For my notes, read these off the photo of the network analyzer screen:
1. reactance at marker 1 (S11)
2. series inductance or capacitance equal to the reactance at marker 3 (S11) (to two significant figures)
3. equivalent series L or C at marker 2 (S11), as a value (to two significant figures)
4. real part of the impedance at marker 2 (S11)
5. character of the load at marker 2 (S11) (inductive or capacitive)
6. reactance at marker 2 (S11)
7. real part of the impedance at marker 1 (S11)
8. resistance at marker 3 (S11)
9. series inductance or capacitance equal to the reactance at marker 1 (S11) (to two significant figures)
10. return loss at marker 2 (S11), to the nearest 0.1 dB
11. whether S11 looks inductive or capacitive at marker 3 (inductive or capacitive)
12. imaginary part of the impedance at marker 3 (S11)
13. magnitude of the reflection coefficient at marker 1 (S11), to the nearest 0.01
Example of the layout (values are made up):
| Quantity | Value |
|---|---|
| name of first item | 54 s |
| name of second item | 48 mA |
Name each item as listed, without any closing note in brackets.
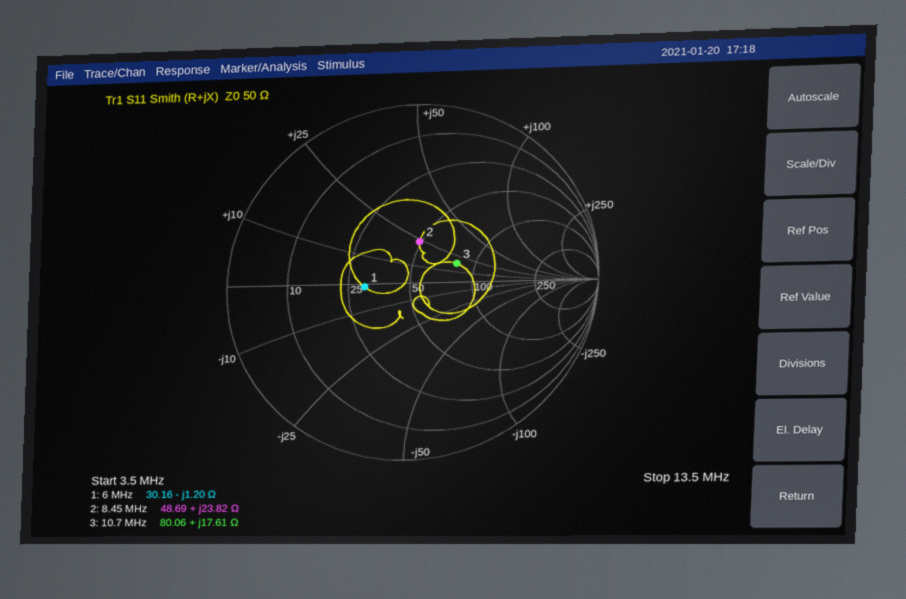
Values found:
| Quantity | Value |
|---|---|
| reactance at marker 1 | -1.20 Ω |
| series inductance or capacitance equal to the reactance at marker 3 (S11) | 260 nH |
| equivalent series L or C at marker 2 (S11), as a value | 450 nH |
| real part of the impedance at marker 2 | 48.69 Ω |
| character of the load at marker 2 (S11) | inductive |
| reactance at marker 2 | +23.82 Ω |
| real part of the impedance at marker 1 | 30.16 Ω |
| resistance at marker 3 | 80.06 Ω |
| series inductance or capacitance equal to the reactance at marker 1 (S11) | 22 nF |
| return loss at marker 2 (S11), to the nearest 0.1 dB | 12.6 dB |
| whether S11 looks inductive or capacitive at marker 3 | inductive |
| imaginary part of the impedance at marker 3 | +17.61 Ω |
| magnitude of the reflection coefficient at marker 1 (S11), to the nearest 0.01 | 0.25 |
